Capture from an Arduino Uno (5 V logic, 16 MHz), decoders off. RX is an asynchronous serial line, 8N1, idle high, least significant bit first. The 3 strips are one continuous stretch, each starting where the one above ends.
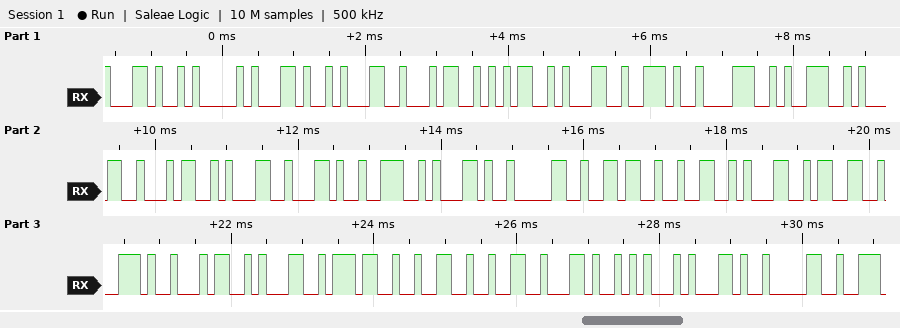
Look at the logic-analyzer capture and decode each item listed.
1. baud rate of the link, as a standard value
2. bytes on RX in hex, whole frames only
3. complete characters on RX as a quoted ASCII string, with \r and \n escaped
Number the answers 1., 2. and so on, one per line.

1. 9600 baud
2. 2C 41 2C 31 34 35 31 2E 38 39 31 34 31 2C 4E 2C 30 36 32 31 33 2E 34 31 37 32 32 2C 45 2C 30
3. ",A,1451.89141,N,06213.41722,E,0"
